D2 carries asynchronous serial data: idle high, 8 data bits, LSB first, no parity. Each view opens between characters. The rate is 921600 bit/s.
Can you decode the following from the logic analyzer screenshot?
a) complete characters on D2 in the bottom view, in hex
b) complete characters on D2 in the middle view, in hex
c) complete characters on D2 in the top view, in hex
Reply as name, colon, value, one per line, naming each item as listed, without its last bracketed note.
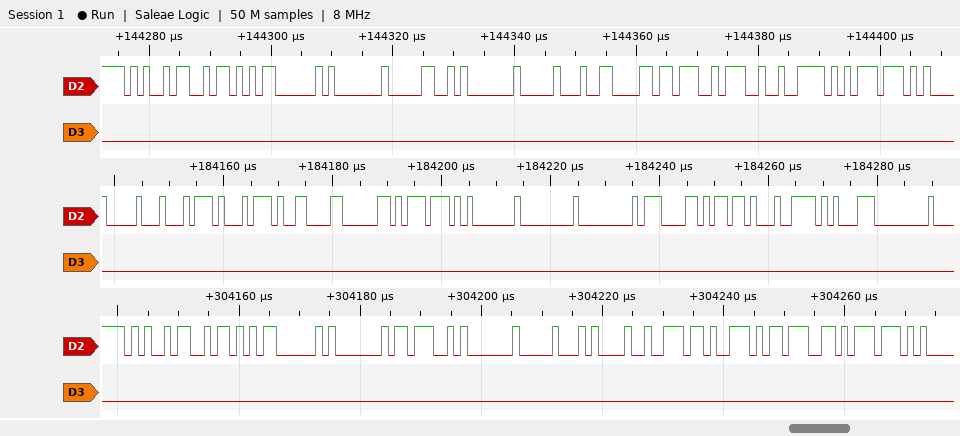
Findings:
complete characters on D2 in the bottom view, in hex: A5, 5A, 03, 01, 3B, 01, 10, 21, 6E, AE, 67, 77
complete characters on D2 in the middle view, in hex: 10, 74, 74, 86, 60, 77, 01, 00, 00, 87, 6D, E4, C5, 00
complete characters on D2 in the top view, in hex: A5, 5A, 03, 01, 30, 01, 10, 86, 3B, 27, 5E, 77
